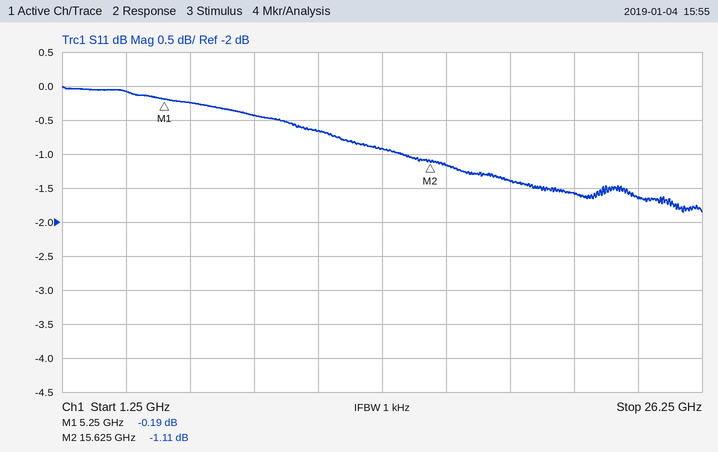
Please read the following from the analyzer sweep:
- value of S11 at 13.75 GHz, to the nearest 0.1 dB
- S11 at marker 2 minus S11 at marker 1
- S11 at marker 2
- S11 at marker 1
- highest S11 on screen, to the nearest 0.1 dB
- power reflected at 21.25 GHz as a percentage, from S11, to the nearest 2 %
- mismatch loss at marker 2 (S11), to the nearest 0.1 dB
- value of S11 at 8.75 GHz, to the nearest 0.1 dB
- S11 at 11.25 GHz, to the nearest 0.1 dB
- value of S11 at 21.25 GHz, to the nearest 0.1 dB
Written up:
-0.9 dB
-0.92 dB
-1.11 dB
-0.19 dB
0.0 dB
70 %
6.5 dB
-0.4 dB
-0.7 dB
-1.6 dB
